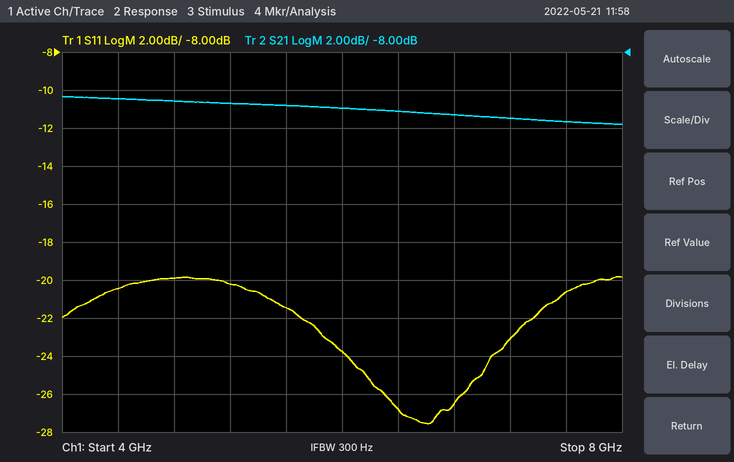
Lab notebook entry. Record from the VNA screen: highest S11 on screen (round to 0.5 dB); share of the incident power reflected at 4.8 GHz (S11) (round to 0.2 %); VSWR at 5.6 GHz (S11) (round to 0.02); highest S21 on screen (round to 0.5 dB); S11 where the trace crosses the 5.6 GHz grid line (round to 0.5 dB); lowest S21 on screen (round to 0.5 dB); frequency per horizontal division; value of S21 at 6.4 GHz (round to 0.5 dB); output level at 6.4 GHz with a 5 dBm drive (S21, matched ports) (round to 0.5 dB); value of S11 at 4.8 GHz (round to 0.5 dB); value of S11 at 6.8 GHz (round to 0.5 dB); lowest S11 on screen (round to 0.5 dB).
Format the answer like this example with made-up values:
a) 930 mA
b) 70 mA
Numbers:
a) -20.0 dB
b) 1.0 %
c) 1.18
d) -10.5 dB
e) -21.5 dB
f) -12.0 dB
g) 400 MHz
h) -11.0 dB
i) -6.0 dBm
j) -20.0 dB
k) -26.5 dB
l) -27.5 dB
